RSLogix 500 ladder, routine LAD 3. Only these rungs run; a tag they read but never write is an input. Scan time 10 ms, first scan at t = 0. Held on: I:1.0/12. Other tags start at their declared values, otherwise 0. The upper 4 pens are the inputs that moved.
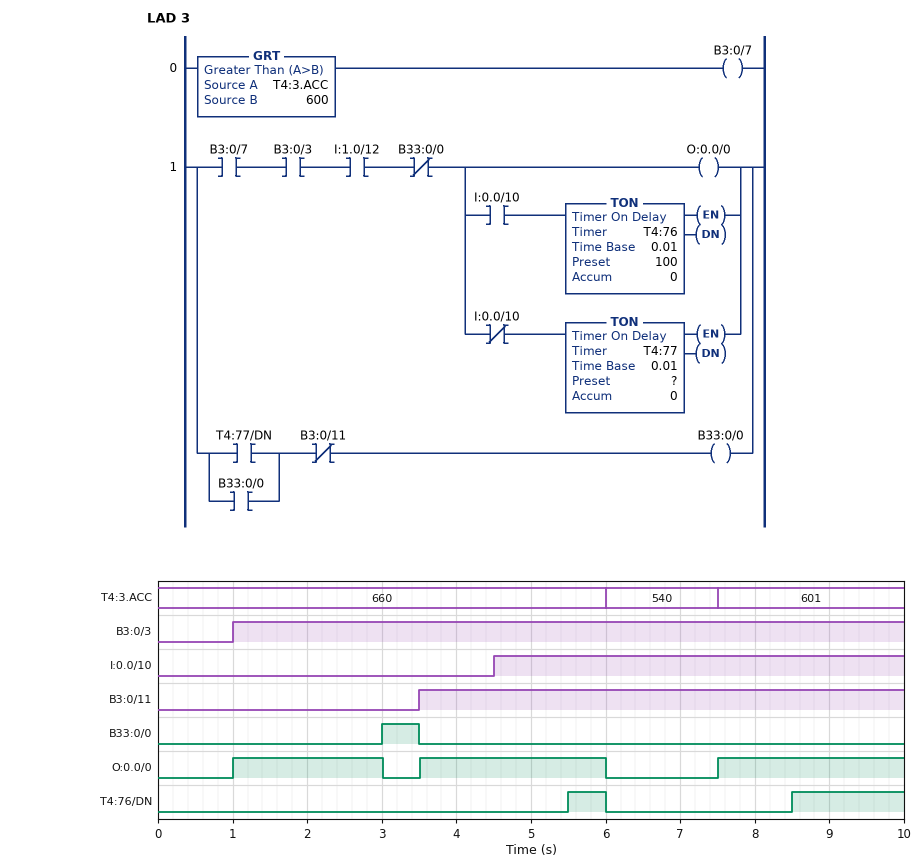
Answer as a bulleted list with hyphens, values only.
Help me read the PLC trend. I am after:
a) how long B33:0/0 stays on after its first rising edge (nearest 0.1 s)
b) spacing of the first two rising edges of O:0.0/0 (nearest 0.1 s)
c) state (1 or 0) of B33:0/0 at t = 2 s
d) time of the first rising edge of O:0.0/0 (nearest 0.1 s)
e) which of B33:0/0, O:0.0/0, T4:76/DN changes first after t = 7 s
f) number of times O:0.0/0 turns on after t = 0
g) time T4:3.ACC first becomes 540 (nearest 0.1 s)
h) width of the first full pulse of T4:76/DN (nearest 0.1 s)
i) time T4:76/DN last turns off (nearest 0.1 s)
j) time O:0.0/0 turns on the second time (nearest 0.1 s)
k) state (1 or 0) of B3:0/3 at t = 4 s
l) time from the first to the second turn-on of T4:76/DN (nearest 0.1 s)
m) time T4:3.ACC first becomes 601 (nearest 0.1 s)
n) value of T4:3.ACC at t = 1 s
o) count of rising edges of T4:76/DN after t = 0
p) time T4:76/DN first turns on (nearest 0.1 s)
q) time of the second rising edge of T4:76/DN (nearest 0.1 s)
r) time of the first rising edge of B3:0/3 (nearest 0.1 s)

- 0.5 s
- 2.5 s
- 0
- 1.0 s
- O:0.0/0
- 3
- 6.0 s
- 0.5 s
- 6.0 s
- 3.5 s
- 1
- 3.0 s
- 7.5 s
- 660
- 2
- 5.5 s
- 8.5 s
- 1.0 s
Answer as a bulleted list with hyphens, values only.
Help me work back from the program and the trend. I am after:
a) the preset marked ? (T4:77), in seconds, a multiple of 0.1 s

- 2.0 s
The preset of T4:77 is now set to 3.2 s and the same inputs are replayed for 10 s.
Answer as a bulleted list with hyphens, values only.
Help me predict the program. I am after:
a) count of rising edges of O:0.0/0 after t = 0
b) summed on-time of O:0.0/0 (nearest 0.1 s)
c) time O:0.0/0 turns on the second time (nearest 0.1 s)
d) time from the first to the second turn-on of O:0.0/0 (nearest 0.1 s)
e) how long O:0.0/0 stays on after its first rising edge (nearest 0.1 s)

- 2
- 7.5 s
- 7.5 s
- 6.5 s
- 5.0 s
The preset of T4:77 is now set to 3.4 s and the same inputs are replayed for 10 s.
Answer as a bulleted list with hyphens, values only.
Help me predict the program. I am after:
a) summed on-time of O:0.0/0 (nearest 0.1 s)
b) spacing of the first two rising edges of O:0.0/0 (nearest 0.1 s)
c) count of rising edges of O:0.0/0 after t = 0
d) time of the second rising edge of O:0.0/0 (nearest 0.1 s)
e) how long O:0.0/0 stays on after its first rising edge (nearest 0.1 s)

- 7.5 s
- 6.5 s
- 2
- 7.5 s
- 5.0 s
